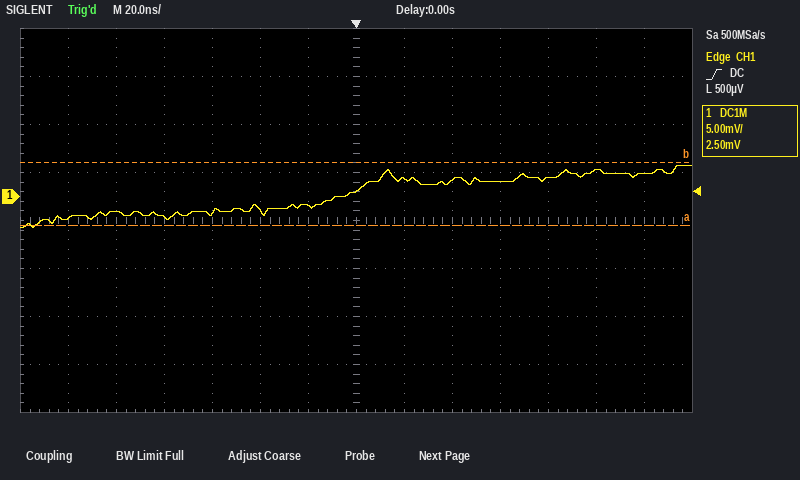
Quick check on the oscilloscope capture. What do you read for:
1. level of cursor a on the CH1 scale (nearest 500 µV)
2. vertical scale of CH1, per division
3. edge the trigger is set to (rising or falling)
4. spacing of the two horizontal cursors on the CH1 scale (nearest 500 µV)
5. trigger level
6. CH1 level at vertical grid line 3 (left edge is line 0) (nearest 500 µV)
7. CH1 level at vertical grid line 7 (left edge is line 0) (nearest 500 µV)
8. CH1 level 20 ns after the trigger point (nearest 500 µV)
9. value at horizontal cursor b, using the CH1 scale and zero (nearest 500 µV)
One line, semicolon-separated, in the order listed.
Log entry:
-3.0 mV; 5 mV; rising; 6.5 mV; 500 µV; -2.0 mV; 500 µV; 2.0 mV; 3.5 mV
